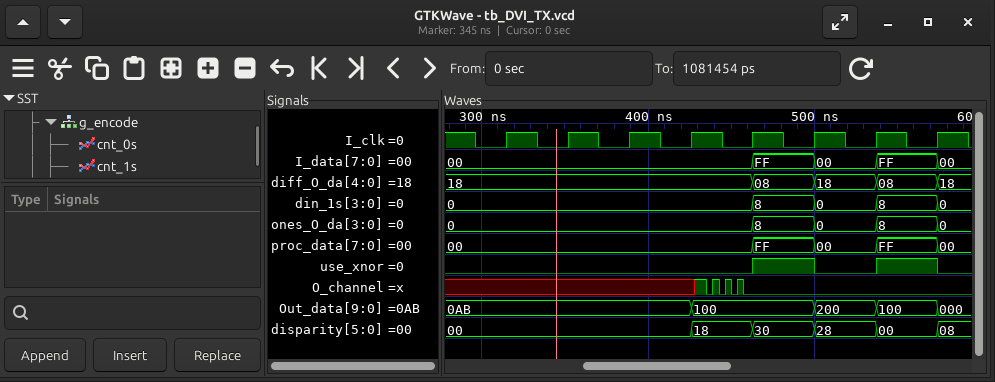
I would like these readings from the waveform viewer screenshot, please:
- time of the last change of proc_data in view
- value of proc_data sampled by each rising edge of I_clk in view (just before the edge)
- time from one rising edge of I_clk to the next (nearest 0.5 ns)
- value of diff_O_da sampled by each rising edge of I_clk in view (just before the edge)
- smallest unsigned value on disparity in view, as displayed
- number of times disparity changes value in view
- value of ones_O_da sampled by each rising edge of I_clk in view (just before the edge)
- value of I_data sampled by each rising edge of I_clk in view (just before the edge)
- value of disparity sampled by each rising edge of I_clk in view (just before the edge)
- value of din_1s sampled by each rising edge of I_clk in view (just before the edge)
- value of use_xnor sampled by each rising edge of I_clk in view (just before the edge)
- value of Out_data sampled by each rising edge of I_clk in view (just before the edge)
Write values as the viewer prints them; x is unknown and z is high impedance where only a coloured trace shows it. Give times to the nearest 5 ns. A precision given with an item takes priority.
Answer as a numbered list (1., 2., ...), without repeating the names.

1. 575 ns
2. 00, 00, 00, 00, 00, FF, 00, FF
3. 37 ns
4. 18, 18, 18, 18, 18, 08, 18, 08
5. 00
6. 5
7. 0, 0, 0, 0, 0, 8, 0, 8
8. 00, 00, 00, 00, 00, FF, 00, FF
9. 00, 00, 00, 00, 18, 30, 28, 00
10. 0, 0, 0, 0, 0, 8, 0, 8
11. 0 0 0 0 0 1 0 1
12. 0AB, 0AB, 0AB, 0AB, 100, 100, 200, 100
